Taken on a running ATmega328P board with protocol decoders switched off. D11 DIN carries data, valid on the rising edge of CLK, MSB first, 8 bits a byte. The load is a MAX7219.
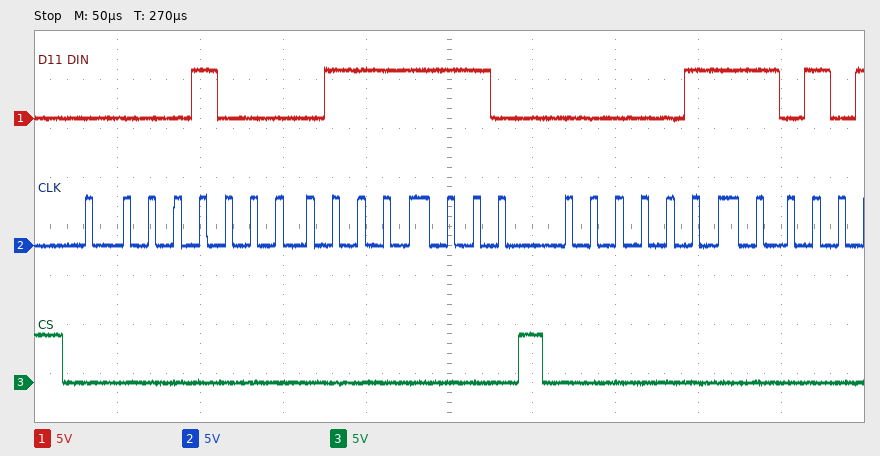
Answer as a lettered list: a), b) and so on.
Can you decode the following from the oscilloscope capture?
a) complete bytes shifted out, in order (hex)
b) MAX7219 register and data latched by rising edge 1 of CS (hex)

a) 08 7E 07
b) register 0x8, data 0x7E
